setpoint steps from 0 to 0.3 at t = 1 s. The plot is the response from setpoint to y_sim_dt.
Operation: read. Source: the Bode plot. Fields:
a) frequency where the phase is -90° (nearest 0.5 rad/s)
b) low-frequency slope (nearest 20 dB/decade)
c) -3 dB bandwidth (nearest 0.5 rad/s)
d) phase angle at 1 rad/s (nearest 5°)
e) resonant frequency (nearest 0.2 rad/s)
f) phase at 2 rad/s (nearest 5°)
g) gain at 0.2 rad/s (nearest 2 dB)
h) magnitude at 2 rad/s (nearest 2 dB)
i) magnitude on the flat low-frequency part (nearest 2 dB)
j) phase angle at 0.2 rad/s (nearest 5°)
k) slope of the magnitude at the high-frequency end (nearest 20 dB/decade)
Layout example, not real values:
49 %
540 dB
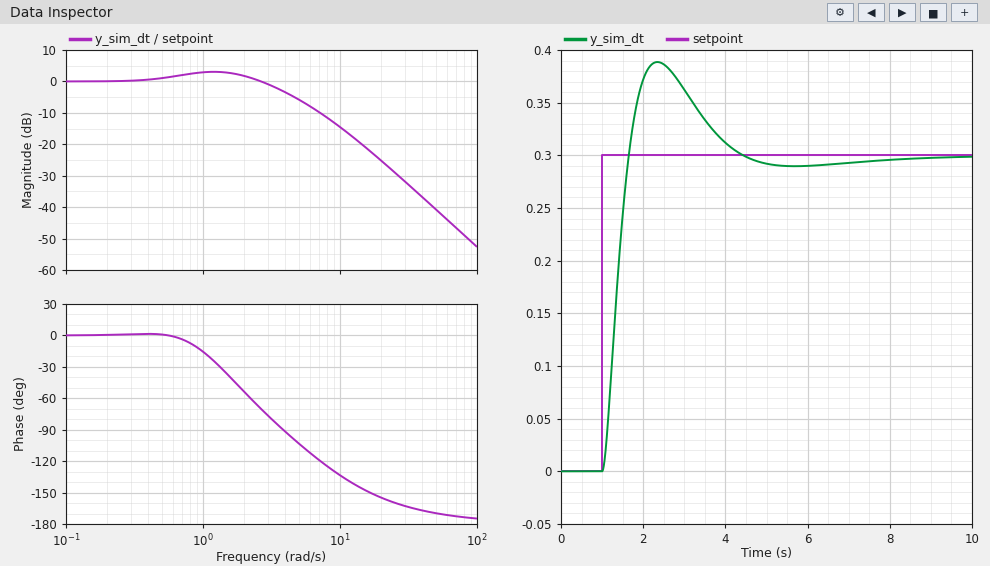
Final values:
4.0 rad/s
0 dB/decade
4.0 rad/s
-15°
1.2 rad/s
-55°
0 dB
2 dB
0 dB
0°
-40 dB/decade
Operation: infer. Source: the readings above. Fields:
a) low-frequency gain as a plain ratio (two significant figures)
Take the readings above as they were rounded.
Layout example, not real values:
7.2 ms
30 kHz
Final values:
1.0
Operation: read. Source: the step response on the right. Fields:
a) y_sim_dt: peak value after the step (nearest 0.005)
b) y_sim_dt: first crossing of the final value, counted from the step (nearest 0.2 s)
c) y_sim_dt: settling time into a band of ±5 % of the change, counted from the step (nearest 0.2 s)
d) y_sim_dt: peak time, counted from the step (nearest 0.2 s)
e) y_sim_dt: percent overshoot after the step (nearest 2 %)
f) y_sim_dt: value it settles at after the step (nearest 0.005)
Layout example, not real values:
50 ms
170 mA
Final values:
0.390
0.6 s
3.0 s
1.4 s
30 %
0.300
